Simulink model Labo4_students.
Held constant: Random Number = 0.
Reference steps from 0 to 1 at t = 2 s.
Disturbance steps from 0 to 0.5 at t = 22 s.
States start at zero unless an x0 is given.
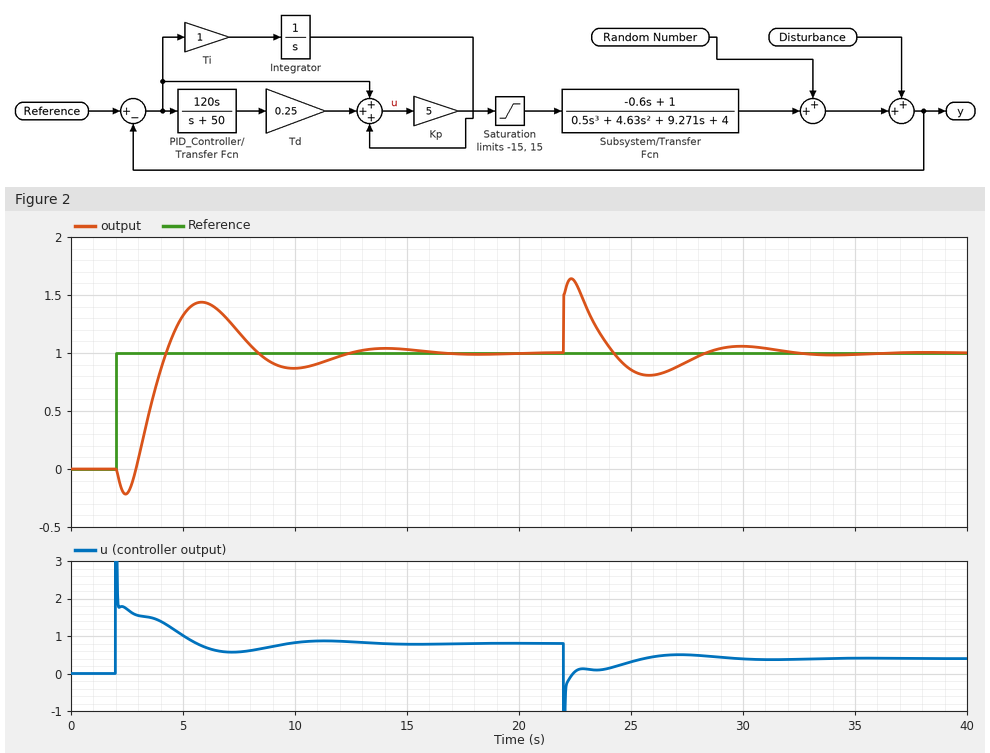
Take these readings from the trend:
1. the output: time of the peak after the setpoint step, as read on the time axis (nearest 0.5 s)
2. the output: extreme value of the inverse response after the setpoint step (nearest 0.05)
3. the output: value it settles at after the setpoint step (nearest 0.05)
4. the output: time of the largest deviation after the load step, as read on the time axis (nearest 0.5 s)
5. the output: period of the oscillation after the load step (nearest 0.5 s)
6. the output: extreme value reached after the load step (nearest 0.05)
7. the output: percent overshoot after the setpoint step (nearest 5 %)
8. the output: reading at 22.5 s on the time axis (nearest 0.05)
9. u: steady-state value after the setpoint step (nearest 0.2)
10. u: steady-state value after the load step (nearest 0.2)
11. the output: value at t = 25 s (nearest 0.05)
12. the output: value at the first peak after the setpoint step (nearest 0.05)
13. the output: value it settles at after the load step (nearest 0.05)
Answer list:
6.0 s
-0.20
1.00
22.5 s
7.5 s
1.65
45 %
1.60
0.8
0.4
0.85
1.45
1.00
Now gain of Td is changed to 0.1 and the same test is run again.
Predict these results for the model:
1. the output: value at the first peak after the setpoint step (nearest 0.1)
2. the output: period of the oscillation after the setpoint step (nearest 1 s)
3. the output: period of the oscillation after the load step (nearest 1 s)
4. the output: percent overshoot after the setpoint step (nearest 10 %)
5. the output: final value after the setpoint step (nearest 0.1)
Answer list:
1.6
7 s
6 s
60 %
1.0
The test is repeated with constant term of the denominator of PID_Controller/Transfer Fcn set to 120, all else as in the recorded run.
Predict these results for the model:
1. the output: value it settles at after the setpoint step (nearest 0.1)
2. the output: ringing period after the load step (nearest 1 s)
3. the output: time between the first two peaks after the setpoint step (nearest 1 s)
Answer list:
1.0
6 s
7 s
